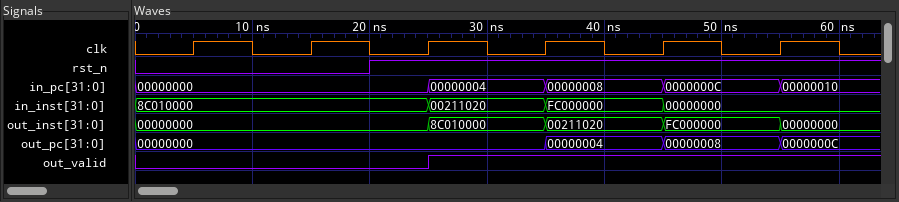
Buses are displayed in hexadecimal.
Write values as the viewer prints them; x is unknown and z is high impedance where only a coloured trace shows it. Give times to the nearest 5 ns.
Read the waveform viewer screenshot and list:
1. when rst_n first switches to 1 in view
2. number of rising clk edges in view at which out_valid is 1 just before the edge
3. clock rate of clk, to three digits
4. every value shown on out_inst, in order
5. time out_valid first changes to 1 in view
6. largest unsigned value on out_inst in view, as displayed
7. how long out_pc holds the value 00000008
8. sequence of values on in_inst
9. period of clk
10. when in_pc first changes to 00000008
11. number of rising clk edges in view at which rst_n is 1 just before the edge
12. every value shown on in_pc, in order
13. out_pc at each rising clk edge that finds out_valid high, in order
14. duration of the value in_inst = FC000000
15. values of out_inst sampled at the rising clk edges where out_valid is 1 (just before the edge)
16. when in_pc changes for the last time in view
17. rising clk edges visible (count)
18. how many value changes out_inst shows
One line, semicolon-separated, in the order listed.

20 ns; 3; 100 MHz; 00000000, 8C010000, 00211020, FC000000, 00000000; 25 ns; FC000000; 10 ns; 8C010000, 00211020, FC000000, 00000000; 10 ns; 35 ns; 4; 00000000, 00000004, 00000008, 0000000C, 00000010; 00000000, 00000004, 00000008; 10 ns; 8C010000, 00211020, FC000000; 55 ns; 6; 4
